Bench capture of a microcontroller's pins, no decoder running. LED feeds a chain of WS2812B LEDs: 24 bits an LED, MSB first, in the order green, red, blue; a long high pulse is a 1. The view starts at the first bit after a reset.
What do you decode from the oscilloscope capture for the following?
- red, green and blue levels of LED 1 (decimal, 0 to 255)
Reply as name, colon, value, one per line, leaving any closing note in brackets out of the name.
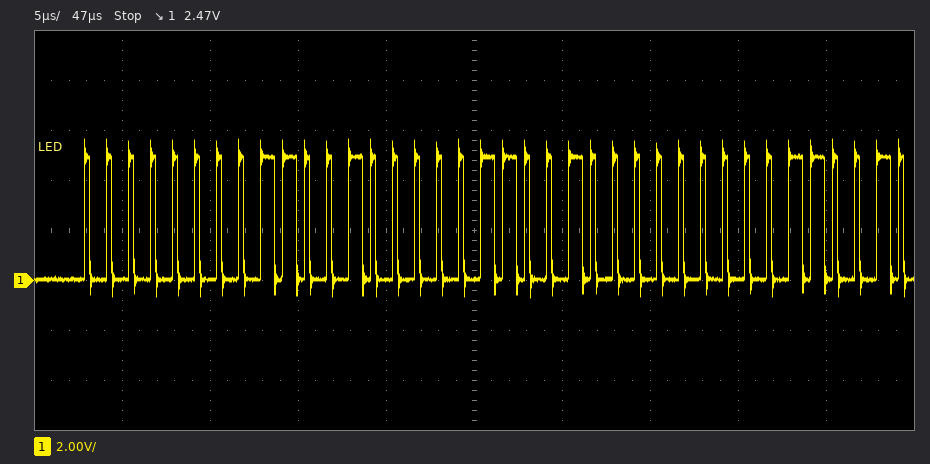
red, green and blue levels of LED 1: 200, 0, 50
